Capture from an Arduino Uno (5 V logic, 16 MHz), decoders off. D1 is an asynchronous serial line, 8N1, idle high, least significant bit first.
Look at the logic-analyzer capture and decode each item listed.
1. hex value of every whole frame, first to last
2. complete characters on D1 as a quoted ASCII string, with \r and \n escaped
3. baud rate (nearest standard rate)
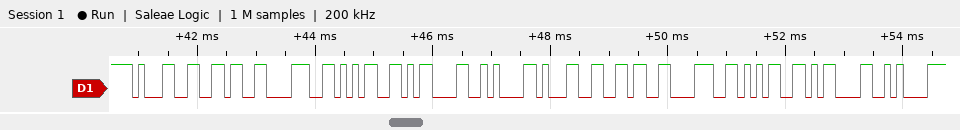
0x31 0x36 0x38 0x35 0x0D 0x0A 0x31 0x36 0x38 0x35 0x0D 0x0A
"1685\r\n1685\r\n"
9600 baud
